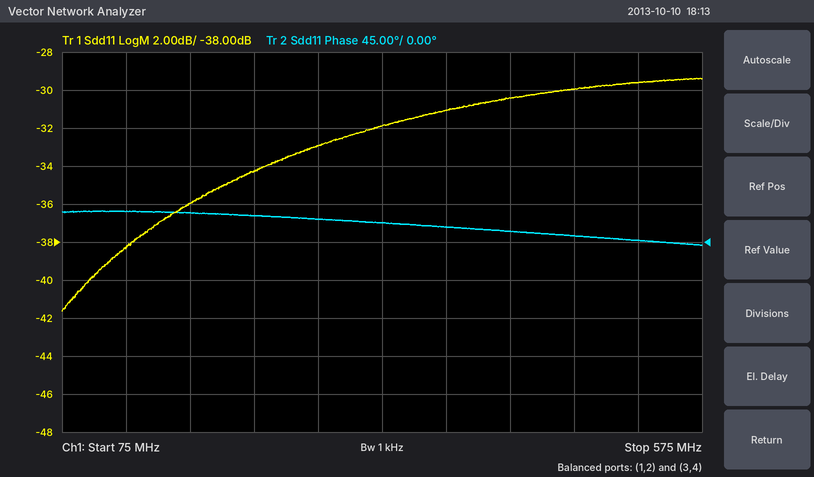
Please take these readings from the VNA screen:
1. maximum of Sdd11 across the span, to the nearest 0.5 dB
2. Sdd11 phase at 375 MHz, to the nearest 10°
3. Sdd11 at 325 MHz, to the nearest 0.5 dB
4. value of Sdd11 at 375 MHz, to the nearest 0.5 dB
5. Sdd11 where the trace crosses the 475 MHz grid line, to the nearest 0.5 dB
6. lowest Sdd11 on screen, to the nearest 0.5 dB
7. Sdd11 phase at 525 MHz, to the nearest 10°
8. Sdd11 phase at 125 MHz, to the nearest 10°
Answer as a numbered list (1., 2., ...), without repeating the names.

1. -29.5 dB
2. 20°
3. -32.0 dB
4. -31.0 dB
5. -30.0 dB
6. -41.5 dB
7. 0°
8. 40°
